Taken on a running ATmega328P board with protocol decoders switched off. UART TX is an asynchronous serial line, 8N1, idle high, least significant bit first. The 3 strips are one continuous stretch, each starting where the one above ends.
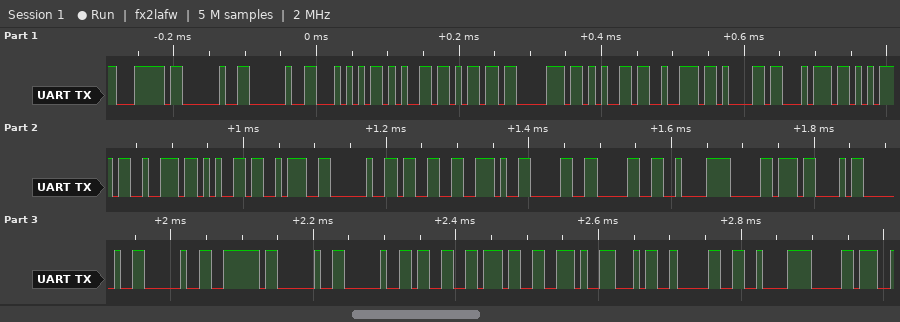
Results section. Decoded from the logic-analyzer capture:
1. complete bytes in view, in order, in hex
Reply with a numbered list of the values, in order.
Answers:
1. 7C 20 20 54 65 6D 70 65 72 61 74 75 72 65 3A 20 33 2E 30 30 C2 B0 43 20 20 7E 20 20 33 37 2E 34 30 C2 B0
